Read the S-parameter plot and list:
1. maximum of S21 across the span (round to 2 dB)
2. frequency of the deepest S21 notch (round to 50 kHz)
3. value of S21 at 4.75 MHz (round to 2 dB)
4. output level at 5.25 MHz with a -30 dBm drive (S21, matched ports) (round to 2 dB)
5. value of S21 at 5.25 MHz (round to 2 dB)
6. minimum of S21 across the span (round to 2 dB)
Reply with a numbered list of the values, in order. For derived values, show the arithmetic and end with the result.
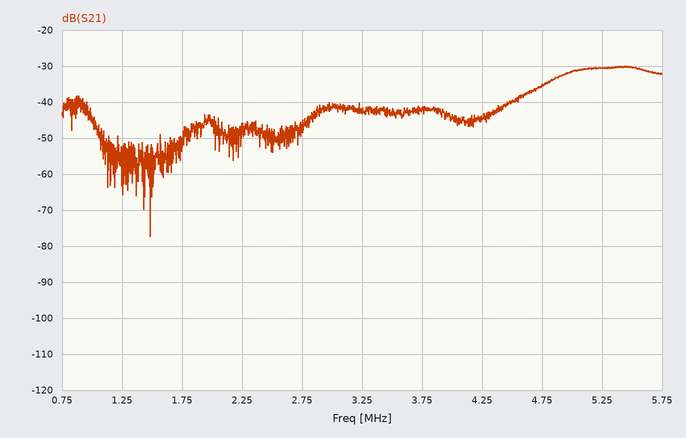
1. -30 dB
2. 1.50 MHz
3. -36 dB
4. -30 dBm + (-30 dB) = -60 dBm
5. -30 dB
6. -78 dB
